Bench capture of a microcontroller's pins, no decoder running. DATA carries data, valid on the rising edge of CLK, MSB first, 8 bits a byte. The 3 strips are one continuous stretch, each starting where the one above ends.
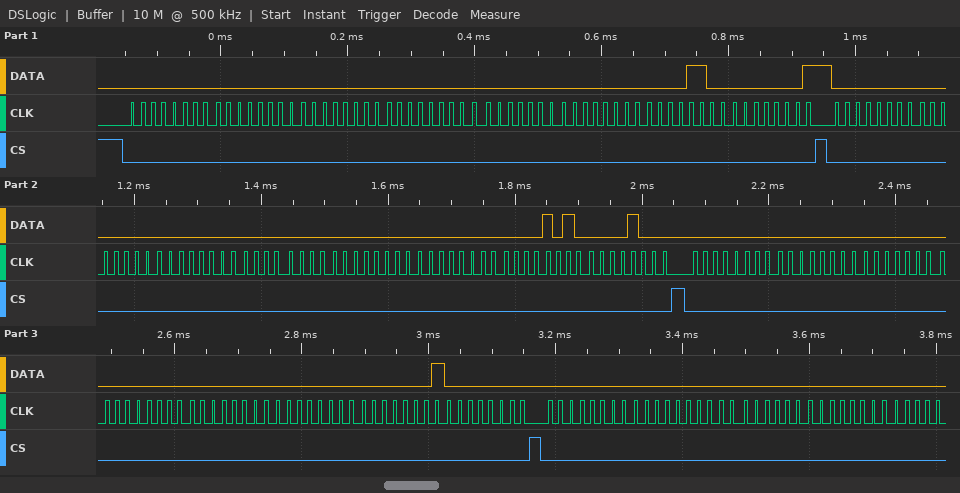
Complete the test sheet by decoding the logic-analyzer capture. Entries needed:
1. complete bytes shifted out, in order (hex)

0x00 0x00 0x00 0x00 0x00 0x00 0x0C 0x01 0x00 0x00 0x00 0x00 0x00 0x00 0x0A 0x08 0x00 0x00 0x00 0x00 0x00 0x00 0x01 0x00 0x00 0x00 0x00 0x00
